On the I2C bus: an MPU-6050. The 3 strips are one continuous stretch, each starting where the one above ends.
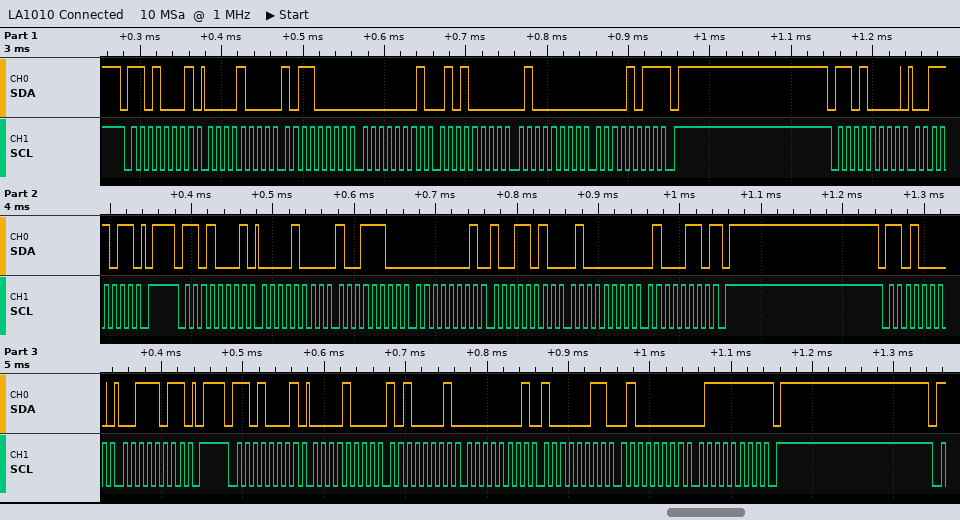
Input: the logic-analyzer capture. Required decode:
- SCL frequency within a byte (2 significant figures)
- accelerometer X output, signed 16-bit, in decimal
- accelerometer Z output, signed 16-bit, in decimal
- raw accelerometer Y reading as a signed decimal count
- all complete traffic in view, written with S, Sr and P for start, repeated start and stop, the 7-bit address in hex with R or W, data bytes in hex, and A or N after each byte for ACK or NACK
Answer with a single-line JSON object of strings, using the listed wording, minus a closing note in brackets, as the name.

{"SCL frequency within a byte": "100 kHz", "accelerometer X output, signed 16-bit, in decimal": "2204", "accelerometer Z output, signed 16-bit, in decimal": "16454", "raw accelerometer Y reading as a signed decimal count": "410", "all complete traffic in view, written with S, Sr and P for start, repeated start and stop, the 7-bit address in hex with R or W, data bytes in hex, and A or N after each byte for ACK or NACK": "S 68R A 08 A B0 A 01 A 50 A 40 A 0B N P S 68W A 3B A P S 68R A 08 A 9C A 01 A 9A A 40 A 46 N P S 68W A 3B A P S 68R A 08 A A1 A 01 A 83 A 40 A 7F N P"}
